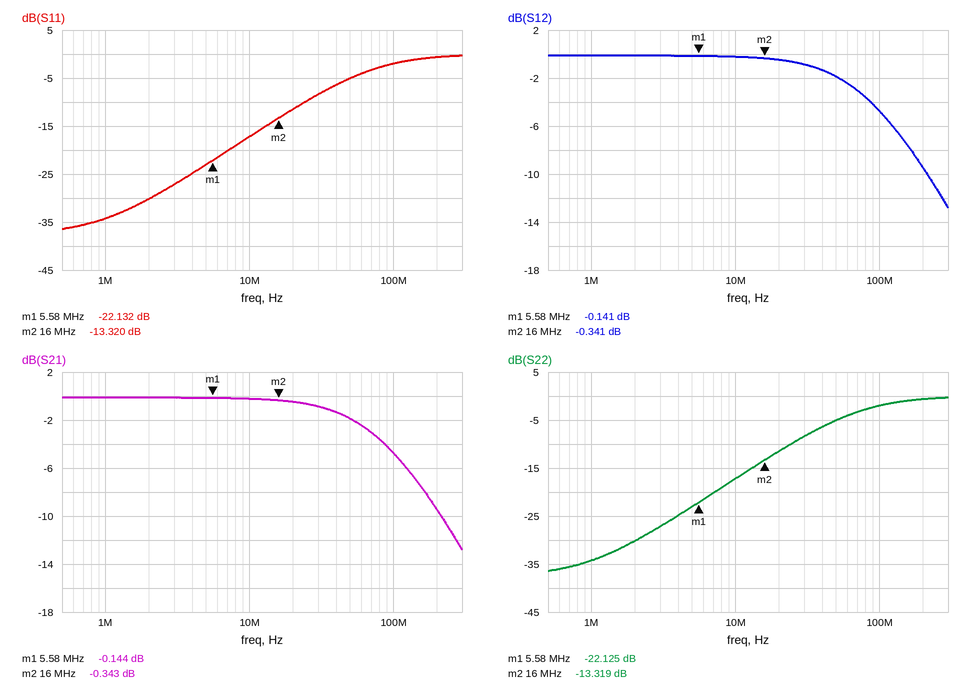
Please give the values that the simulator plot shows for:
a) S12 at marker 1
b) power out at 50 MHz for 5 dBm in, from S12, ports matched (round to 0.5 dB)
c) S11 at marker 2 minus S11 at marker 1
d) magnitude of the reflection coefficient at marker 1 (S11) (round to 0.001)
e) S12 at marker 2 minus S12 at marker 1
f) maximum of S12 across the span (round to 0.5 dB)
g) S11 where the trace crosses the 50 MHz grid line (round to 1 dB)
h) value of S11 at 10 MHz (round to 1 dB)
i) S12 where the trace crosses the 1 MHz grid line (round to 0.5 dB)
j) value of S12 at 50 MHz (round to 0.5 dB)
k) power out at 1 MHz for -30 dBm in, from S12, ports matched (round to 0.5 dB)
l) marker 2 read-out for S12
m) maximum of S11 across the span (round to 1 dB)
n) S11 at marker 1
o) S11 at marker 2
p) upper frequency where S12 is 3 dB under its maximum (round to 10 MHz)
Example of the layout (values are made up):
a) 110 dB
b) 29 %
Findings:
a) -0.141 dB
b) 3.0 dBm
c) 8.812 dB
d) 0.078
e) -0.200 dB
f) 0.0 dB
g) -5 dB
h) -17 dB
i) 0.0 dB
j) -2.0 dB
k) -30.0 dBm
l) -0.341 dB
m) 0 dB
n) -22.132 dB
o) -13.320 dB
p) 70 MHz
